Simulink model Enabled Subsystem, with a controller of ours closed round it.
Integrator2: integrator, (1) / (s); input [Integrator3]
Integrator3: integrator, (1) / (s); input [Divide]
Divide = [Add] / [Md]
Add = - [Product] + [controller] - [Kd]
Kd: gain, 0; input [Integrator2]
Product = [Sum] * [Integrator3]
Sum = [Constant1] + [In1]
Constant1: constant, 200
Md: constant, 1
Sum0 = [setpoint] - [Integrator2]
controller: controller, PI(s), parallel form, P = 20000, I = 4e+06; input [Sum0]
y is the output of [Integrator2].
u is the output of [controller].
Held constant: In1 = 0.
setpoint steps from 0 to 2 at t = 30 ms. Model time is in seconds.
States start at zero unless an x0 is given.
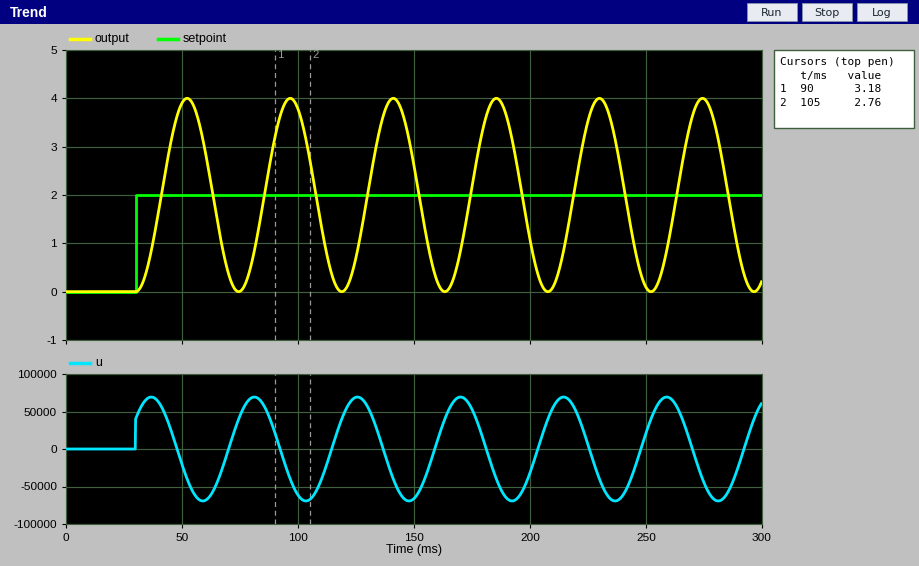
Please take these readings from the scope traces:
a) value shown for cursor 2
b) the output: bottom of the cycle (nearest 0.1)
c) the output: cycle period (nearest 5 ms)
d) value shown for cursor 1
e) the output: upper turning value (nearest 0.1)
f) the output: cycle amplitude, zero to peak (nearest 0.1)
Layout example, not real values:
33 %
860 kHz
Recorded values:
2.76
0.0
45 ms
3.18
4.0
2.0
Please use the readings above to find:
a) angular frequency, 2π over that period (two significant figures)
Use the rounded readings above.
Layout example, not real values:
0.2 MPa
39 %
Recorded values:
0.14 rad/ms
